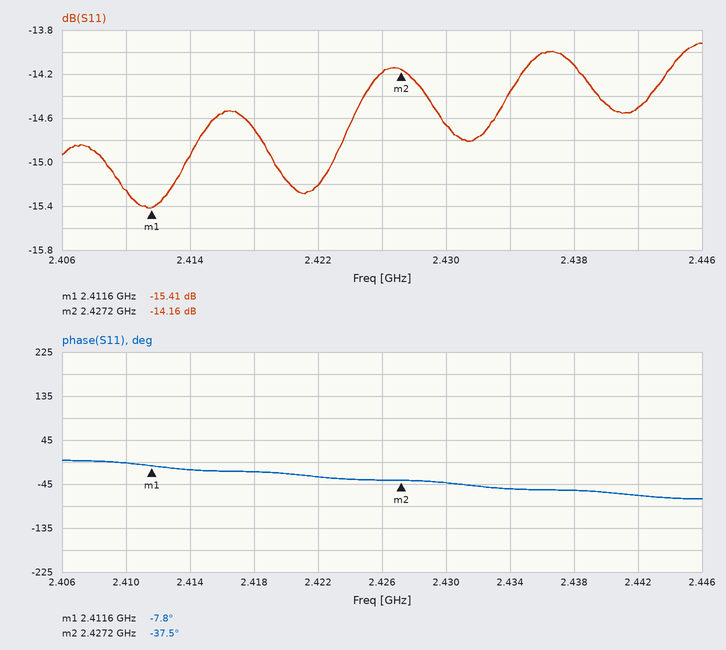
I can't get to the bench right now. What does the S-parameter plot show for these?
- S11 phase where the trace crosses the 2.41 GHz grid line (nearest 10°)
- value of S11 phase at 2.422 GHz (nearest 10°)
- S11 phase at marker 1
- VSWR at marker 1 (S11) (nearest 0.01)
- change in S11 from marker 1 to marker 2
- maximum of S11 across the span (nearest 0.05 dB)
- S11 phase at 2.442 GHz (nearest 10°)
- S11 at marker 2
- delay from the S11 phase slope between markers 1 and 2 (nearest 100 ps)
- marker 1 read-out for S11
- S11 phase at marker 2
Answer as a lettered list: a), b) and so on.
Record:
a) 0°
b) -30°
c) -7.8°
d) 1.41
e) 1.25 dB
f) -13.90 dB
g) -70°
h) -14.16 dB
i) 5.3 ns
j) -15.41 dB
k) -37.5°
